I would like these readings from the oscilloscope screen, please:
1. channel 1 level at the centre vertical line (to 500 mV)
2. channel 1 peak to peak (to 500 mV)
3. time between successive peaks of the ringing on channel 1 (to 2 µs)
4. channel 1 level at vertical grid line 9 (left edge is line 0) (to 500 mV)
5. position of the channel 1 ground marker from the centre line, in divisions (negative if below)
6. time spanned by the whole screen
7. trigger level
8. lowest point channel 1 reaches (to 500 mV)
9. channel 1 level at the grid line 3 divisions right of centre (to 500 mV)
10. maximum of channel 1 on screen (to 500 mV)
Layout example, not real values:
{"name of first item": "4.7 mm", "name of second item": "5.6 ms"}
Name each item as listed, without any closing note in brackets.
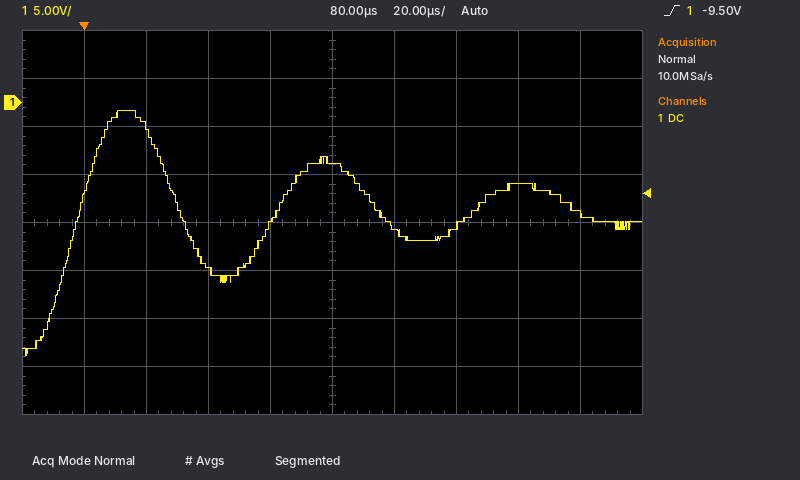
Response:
{"channel 1 level at the centre vertical line": "-6.5 V", "channel 1 peak to peak": "25.5 V", "time between successive peaks of the ringing on channel 1": "64 µs", "channel 1 level at vertical grid line 9 (left edge is line 0)": "-11.5 V", "position of the channel 1 ground marker from the centre line, in divisions": "+2.5 div", "time spanned by the whole screen": "200 µs", "trigger level": "-9.50 V", "lowest point channel 1 reaches": "-26.5 V", "channel 1 level at the grid line 3 divisions right of centre": "-8.5 V", "maximum of channel 1 on screen": "-1.0 V"}
